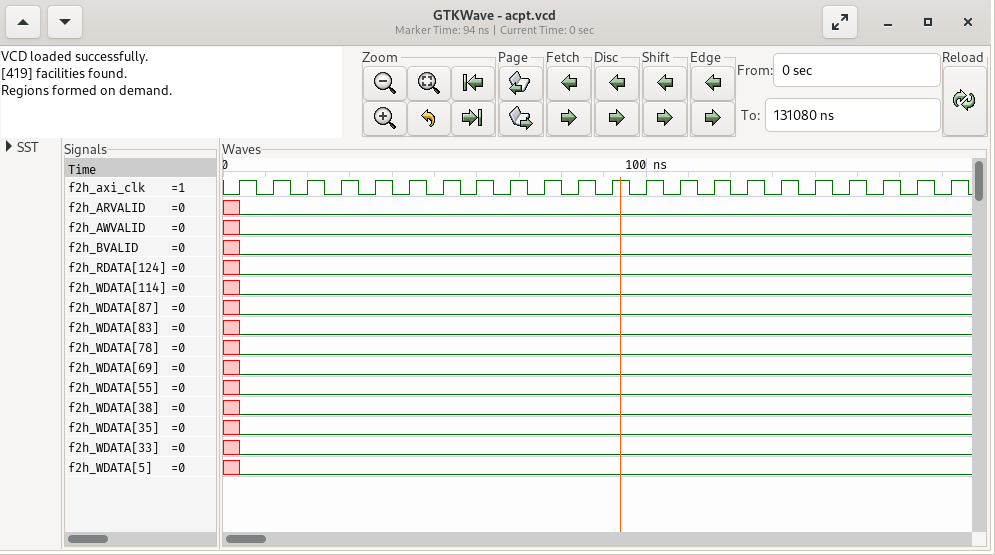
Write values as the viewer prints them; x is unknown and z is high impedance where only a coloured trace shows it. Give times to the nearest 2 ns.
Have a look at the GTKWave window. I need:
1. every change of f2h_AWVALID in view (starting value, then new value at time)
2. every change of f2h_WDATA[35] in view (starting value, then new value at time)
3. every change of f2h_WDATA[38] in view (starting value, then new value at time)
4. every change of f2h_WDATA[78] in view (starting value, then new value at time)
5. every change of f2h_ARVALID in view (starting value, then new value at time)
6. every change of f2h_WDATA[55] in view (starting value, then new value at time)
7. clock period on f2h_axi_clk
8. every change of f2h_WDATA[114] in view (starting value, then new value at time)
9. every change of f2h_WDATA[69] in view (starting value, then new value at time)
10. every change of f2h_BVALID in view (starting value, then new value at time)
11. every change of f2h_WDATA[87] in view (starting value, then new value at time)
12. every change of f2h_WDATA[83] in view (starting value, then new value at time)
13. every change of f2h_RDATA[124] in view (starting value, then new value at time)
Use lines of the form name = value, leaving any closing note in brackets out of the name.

every change of f2h_AWVALID in view = x, 0 at 4 ns
every change of f2h_WDATA[35] in view = x, 0 at 4 ns
every change of f2h_WDATA[38] in view = x, 0 at 4 ns
every change of f2h_WDATA[78] in view = x, 0 at 4 ns
every change of f2h_ARVALID in view = x, 0 at 4 ns
every change of f2h_WDATA[55] in view = x, 0 at 4 ns
clock period on f2h_axi_clk = 8 ns
every change of f2h_WDATA[114] in view = x, 0 at 4 ns
every change of f2h_WDATA[69] in view = x, 0 at 4 ns
every change of f2h_BVALID in view = x, 0 at 4 ns
every change of f2h_WDATA[87] in view = x, 0 at 4 ns
every change of f2h_WDATA[83] in view = x, 0 at 4 ns
every change of f2h_RDATA[124] in view = x, 0 at 4 ns
